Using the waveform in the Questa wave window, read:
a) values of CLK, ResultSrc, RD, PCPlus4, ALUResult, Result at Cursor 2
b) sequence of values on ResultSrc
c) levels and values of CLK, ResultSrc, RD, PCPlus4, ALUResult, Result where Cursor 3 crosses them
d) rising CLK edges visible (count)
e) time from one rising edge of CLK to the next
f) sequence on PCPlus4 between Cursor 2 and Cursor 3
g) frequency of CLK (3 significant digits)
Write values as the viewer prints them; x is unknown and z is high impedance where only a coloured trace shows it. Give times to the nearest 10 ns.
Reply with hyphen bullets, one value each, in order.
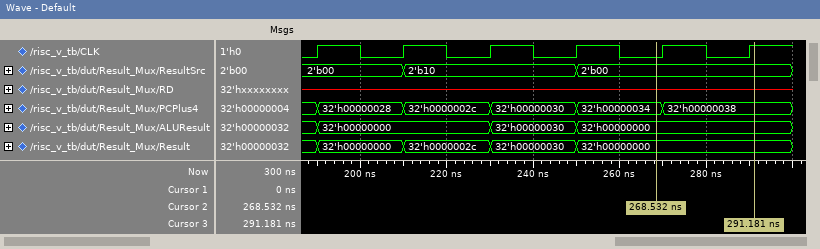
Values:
- CLK=0, ResultSrc=2'b00, RD=x, PCPlus4=32'h00000034, ALUResult=32'h00000000, Result=32'h00000000
- 2'b00, 2'b10, 2'b00
- CLK=1, ResultSrc=2'b00, RD=x, PCPlus4=32'h00000038, ALUResult=32'h00000000, Result=32'h00000000
- 6
- 20 ns
- 32'h00000034, 32'h00000038
- 50.0 MHz
